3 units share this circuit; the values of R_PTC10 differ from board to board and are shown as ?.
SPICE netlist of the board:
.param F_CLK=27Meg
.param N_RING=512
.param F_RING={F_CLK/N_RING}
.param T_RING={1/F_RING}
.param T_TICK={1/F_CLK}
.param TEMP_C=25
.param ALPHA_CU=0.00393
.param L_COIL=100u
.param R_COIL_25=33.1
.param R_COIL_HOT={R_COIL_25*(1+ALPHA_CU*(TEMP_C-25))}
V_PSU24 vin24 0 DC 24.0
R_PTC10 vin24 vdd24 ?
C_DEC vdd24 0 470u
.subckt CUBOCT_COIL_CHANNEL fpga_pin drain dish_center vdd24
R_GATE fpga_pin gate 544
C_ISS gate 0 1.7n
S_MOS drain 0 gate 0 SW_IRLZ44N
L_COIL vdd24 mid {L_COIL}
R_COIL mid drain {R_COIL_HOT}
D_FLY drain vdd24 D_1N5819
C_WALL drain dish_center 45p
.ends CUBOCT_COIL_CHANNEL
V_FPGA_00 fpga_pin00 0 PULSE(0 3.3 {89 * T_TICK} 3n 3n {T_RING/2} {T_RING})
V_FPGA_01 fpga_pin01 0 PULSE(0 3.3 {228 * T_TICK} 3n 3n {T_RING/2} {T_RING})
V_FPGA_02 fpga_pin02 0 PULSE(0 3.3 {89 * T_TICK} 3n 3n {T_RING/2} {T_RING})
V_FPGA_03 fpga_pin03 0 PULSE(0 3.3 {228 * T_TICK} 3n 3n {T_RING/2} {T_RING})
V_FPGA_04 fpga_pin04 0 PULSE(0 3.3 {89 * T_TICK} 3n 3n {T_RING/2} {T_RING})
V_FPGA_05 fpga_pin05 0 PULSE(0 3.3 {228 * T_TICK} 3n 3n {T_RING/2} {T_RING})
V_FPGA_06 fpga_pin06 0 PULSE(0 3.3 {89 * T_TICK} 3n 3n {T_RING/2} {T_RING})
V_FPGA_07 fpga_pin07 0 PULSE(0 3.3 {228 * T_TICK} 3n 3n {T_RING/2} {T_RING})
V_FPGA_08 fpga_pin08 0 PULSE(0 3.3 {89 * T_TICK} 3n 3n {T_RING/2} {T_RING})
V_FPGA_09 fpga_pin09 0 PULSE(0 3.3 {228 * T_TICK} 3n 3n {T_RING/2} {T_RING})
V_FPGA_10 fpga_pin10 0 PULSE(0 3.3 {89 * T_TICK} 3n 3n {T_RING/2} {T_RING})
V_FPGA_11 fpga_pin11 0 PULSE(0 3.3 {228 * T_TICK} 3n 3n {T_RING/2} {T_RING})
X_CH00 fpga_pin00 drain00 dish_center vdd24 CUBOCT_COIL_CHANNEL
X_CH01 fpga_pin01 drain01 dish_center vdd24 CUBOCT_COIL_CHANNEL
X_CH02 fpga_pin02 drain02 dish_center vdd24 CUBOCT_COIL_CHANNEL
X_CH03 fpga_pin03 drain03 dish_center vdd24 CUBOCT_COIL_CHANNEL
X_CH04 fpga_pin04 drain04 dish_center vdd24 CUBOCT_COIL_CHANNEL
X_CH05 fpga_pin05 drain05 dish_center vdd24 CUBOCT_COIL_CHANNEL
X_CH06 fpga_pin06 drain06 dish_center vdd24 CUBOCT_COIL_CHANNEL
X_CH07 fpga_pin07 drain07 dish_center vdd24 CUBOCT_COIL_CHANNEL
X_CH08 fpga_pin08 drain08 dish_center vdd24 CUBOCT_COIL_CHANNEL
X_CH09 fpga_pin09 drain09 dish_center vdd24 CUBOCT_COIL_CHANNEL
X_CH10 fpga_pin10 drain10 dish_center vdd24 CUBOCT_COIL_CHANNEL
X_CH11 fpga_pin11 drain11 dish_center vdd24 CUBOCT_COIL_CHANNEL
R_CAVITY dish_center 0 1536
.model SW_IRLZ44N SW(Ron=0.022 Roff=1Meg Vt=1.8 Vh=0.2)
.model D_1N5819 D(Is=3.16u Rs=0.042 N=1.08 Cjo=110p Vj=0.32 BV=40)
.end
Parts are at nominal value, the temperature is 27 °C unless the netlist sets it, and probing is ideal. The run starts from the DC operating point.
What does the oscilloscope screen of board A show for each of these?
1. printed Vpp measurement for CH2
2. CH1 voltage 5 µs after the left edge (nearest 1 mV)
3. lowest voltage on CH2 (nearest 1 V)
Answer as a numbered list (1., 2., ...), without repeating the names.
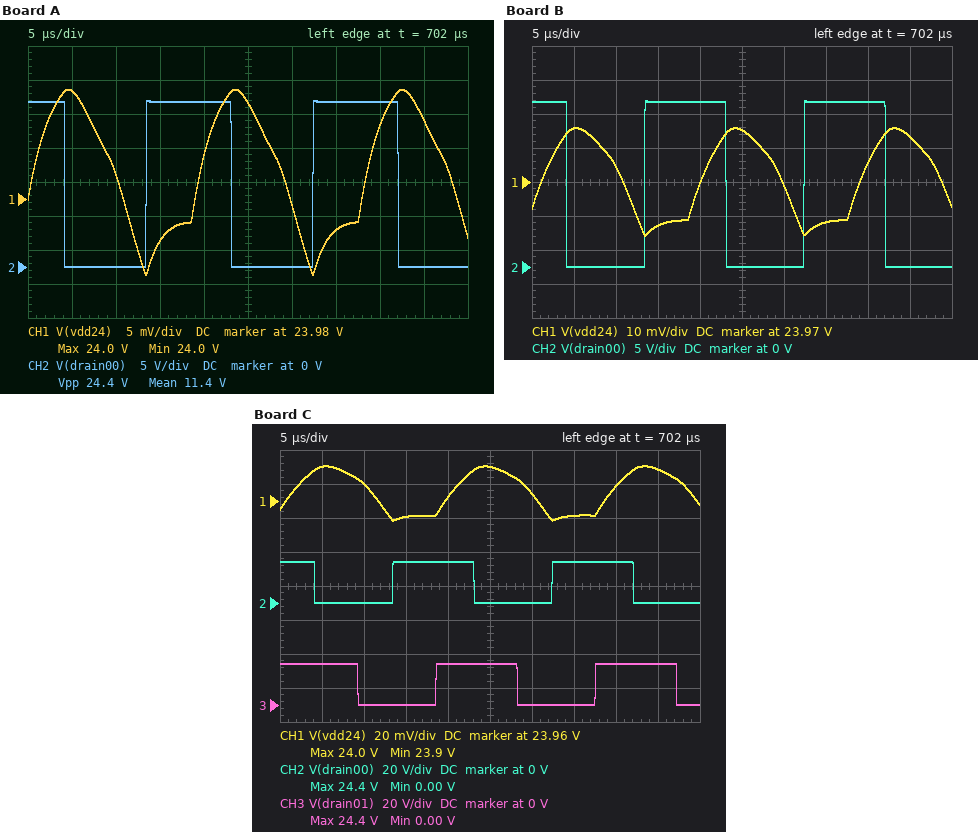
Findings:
1. 24.4 V
2. 23.996 V
3. 0 V
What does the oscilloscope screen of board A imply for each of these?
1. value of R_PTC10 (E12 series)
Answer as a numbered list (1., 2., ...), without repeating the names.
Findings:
1. 5.6 mΩ
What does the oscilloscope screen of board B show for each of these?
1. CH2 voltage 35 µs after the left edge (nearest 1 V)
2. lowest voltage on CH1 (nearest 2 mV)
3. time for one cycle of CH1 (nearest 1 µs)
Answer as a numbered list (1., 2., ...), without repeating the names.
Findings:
1. 24 V
2. 23.954 V
3. 19 µs
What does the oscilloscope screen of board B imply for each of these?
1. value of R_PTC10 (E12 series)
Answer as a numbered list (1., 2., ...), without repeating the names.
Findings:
1. 0.01 Ω
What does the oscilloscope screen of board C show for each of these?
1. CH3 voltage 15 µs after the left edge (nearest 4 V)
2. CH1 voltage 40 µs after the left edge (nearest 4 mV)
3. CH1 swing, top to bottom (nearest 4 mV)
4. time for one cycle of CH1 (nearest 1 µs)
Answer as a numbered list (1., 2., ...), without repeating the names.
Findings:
1. 0 V
2. 23.968 V
3. 32 mV
4. 19 µs
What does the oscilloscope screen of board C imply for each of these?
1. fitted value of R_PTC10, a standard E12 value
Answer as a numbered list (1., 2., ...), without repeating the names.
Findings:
1. 0.012 Ω
